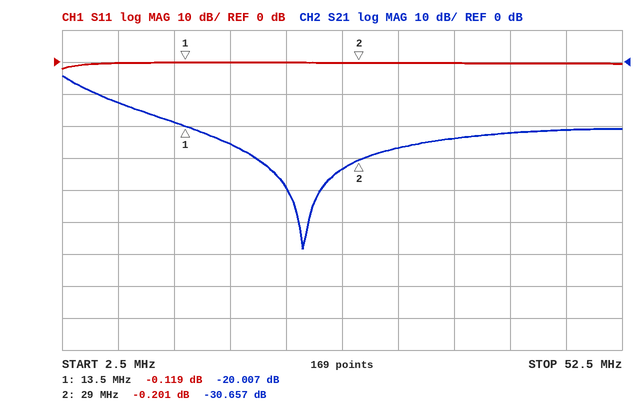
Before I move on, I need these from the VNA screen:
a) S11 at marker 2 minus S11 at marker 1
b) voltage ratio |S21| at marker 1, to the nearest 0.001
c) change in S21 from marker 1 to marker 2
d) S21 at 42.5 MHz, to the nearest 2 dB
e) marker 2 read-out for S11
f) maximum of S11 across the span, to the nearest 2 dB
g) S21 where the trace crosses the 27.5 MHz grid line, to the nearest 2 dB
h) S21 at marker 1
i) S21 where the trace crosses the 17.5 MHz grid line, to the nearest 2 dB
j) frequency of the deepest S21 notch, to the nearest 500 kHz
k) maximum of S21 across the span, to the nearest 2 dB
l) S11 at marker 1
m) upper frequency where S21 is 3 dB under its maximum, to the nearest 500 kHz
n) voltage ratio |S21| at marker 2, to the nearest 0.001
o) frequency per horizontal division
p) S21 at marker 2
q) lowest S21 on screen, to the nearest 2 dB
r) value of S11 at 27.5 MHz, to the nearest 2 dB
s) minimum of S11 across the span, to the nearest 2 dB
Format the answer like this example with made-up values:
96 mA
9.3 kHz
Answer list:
-0.082 dB
0.100
-10.650 dB
-22 dB
-0.201 dB
0 dB
-34 dB
-20.007 dB
-26 dB
24.0 MHz
-4 dB
-0.119 dB
4.0 MHz
0.029
5 MHz
-30.657 dB
-58 dB
0 dB
-2 dB
